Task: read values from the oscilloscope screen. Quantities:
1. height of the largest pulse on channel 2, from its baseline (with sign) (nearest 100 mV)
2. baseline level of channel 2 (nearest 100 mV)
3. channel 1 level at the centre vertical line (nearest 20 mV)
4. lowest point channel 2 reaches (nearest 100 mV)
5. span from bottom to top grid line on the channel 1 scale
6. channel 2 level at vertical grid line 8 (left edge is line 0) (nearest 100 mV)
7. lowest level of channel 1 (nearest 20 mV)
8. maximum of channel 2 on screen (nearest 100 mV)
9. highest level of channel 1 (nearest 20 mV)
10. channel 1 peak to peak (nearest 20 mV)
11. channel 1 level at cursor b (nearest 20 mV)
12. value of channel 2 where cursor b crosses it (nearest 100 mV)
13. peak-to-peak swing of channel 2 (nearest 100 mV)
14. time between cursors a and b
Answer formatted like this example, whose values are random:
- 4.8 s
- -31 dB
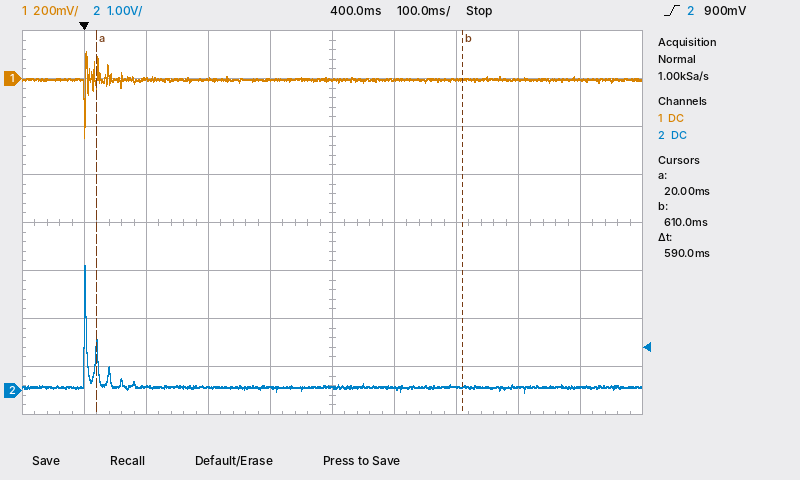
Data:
- +2.5 V
- 100 mV
- 0 mV
- 0.0 V
- 1.6 V
- 100 mV
- -240 mV
- 2.6 V
- 120 mV
- 360 mV
- 0 mV
- 100 mV
- 2.6 V
- 590 ms
